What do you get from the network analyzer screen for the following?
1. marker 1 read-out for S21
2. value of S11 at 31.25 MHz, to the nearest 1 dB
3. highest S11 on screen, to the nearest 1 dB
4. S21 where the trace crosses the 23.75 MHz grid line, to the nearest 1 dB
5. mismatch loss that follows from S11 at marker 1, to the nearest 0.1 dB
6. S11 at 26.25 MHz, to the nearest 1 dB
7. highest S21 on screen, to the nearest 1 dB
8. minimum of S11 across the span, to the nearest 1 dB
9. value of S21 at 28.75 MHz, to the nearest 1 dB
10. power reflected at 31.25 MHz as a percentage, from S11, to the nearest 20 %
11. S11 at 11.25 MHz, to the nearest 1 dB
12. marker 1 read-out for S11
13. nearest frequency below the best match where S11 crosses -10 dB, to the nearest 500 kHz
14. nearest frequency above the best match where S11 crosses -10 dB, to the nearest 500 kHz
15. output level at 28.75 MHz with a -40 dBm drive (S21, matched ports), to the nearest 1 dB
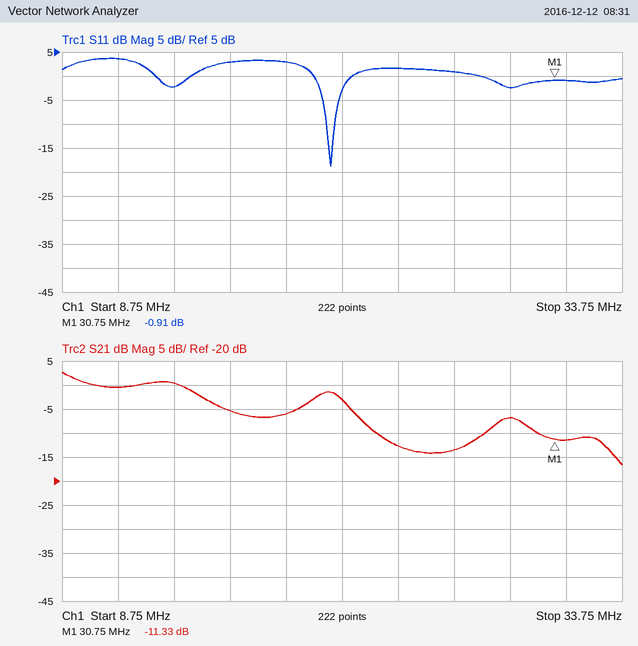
-11.33 dB
-1 dB
4 dB
-13 dB
7.2 dB
1 dB
3 dB
-19 dB
-7 dB
80 %
4 dB
-0.91 dB
20.5 MHz
21.0 MHz
-47 dBm
